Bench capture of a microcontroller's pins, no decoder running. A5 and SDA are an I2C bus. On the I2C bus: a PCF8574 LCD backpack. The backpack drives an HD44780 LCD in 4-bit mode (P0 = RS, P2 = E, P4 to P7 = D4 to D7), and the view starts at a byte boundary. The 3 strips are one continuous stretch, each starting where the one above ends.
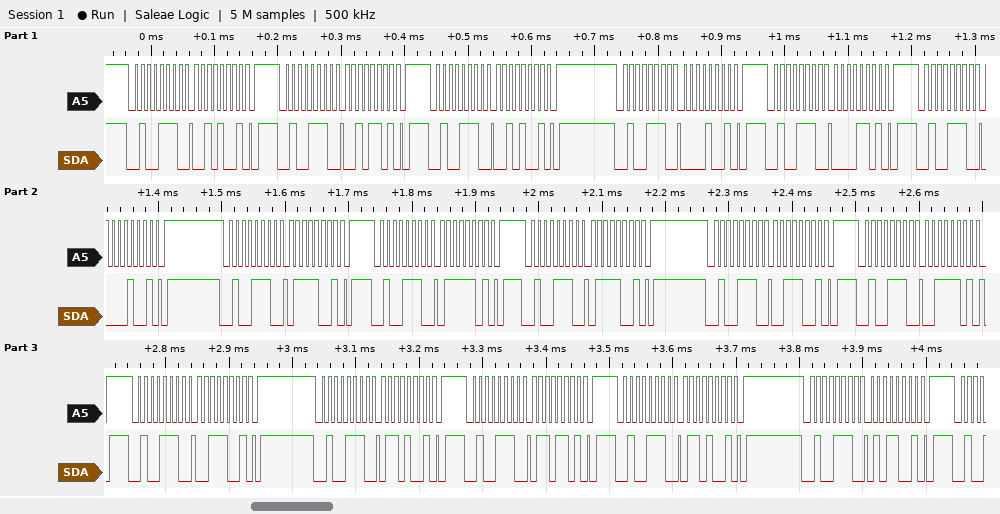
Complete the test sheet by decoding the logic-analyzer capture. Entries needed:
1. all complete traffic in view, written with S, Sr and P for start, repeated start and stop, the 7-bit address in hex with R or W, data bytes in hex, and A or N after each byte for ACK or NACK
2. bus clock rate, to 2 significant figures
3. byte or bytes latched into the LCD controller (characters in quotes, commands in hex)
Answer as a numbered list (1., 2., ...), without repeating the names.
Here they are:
1. S 27W A 29 A P S 27W A 2D A P S 27W A 29 A P S 27W A 09 A P S 27W A 0D A P S 27W A 09 A P S 27W A 79 A P S 27W A 7D A P S 27W A 79 A P S 27W A 39 A P S 27W A 3D A P S 27W A 39 A P S 27W A 69 A P S 27W A 6D A P S 27W A 69 A P S 27W A 59 A P
2. 100 kHz
3. ' ' 's'
